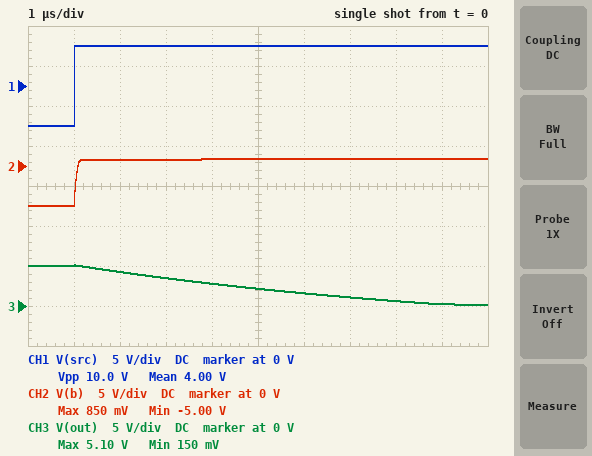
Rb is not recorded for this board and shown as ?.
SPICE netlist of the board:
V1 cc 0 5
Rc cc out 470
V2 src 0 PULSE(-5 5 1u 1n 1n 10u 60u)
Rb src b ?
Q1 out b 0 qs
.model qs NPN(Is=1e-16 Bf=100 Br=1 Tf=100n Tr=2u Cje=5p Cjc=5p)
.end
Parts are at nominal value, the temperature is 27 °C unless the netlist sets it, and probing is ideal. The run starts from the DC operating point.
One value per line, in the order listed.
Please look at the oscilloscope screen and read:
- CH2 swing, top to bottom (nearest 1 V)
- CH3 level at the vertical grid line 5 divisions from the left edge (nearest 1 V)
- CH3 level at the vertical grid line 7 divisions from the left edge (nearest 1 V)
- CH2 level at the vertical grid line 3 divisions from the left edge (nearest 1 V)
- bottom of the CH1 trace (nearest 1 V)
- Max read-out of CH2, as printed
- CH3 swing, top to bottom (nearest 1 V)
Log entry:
6 V
2 V
1 V
1 V
-5 V
850 mV
5 V
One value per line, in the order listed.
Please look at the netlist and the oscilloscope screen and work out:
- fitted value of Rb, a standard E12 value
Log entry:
22 kΩ
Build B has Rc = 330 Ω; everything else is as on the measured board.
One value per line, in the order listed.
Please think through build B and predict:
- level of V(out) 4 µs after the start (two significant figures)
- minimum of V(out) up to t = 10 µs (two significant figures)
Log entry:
3.4 V
1.3 V
